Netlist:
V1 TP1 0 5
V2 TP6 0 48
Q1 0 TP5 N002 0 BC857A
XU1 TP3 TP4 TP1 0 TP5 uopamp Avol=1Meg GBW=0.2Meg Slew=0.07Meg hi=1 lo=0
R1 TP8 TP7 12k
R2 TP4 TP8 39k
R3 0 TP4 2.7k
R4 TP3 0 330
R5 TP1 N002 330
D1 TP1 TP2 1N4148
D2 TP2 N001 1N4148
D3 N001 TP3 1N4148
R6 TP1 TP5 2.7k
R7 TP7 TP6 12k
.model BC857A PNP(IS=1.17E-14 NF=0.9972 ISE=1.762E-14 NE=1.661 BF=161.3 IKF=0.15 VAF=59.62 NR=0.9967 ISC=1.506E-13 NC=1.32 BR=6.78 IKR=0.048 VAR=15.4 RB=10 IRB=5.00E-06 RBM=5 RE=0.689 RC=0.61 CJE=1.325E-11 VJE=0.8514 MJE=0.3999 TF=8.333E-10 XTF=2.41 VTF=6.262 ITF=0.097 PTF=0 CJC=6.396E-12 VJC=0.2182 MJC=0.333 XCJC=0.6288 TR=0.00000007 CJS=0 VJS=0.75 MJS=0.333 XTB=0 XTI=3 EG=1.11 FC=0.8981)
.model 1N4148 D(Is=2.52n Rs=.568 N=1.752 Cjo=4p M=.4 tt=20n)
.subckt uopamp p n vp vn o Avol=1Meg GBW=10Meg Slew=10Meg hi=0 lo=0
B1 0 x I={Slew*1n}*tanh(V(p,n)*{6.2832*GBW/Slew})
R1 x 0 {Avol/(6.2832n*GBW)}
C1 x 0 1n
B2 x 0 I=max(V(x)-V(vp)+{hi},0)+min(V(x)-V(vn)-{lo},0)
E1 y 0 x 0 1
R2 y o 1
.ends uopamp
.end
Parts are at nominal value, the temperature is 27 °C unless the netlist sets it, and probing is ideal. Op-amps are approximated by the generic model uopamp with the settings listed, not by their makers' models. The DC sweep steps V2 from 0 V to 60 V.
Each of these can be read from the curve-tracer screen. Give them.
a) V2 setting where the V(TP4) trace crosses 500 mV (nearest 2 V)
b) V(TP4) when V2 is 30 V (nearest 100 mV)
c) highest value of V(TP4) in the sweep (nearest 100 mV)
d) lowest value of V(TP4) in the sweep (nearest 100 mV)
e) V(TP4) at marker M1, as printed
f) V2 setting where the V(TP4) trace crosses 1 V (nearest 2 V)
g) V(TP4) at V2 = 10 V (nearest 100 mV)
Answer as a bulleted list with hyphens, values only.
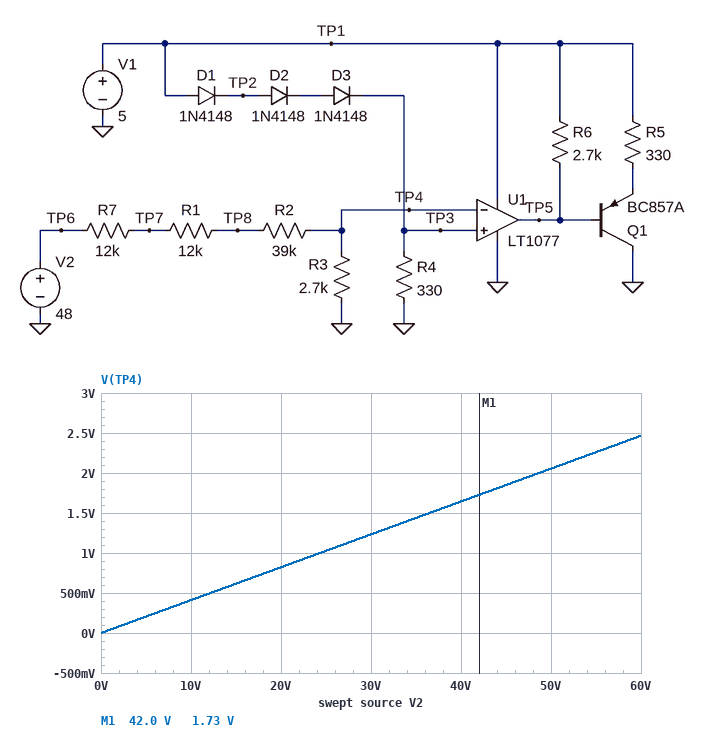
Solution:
- 12 V
- 1.2 V
- 2.5 V
- 0 V
- 1.73 V
- 24 V
- 400 mV
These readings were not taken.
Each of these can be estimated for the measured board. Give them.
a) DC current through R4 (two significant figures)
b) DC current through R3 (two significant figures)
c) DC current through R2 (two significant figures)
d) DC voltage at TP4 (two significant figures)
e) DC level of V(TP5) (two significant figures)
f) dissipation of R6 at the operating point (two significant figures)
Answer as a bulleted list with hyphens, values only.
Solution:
- 8.9 mA
- 730 µA
- 730 µA
- 2.0 V
- 4.0 V
- 370 µW
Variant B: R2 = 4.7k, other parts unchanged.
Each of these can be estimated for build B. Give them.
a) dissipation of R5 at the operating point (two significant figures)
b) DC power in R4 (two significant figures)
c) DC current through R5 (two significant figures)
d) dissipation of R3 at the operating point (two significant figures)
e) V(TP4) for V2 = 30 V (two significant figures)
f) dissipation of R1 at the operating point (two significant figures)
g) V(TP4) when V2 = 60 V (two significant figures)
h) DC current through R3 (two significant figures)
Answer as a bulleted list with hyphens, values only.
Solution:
- 55 mW
- 26 mW
- 13 mA
- 6.3 mW
- 2.6 V
- 28 mW
- 5.2 V
- 1.5 mA
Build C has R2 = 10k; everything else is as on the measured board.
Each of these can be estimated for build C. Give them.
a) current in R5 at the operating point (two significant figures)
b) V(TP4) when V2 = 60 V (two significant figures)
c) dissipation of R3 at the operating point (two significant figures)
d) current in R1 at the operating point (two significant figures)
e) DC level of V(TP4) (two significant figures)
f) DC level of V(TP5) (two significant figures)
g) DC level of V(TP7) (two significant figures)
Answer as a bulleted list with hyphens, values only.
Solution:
- 13 mA
- 4.4 V
- 4.6 mW
- 1.3 mA
- 3.5 V
- 1.9 mV
- 32 V
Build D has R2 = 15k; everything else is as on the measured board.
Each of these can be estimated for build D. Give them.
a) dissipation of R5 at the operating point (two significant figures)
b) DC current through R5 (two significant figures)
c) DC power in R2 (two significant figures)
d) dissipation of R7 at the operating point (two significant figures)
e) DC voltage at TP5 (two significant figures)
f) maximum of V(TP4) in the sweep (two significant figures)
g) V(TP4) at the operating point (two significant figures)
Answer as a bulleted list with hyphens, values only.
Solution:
- 55 mW
- 13 mA
- 20 mW
- 16 mW
- 1.9 mV
- 3.9 V
- 3.1 V
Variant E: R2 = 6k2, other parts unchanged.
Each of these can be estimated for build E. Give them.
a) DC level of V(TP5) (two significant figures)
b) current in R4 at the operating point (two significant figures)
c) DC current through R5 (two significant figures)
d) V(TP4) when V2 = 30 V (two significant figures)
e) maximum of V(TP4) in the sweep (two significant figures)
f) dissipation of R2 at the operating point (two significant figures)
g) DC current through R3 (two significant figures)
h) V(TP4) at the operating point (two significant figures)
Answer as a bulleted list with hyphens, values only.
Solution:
- 1.9 mV
- 8.9 mA
- 13 mA
- 2.5 V
- 4.9 V
- 13 mW
- 1.5 mA
- 3.9 V
